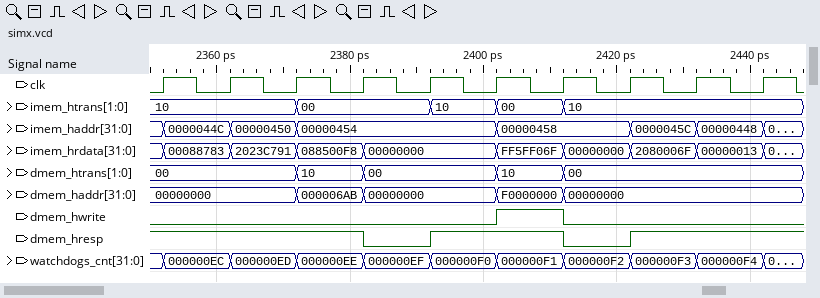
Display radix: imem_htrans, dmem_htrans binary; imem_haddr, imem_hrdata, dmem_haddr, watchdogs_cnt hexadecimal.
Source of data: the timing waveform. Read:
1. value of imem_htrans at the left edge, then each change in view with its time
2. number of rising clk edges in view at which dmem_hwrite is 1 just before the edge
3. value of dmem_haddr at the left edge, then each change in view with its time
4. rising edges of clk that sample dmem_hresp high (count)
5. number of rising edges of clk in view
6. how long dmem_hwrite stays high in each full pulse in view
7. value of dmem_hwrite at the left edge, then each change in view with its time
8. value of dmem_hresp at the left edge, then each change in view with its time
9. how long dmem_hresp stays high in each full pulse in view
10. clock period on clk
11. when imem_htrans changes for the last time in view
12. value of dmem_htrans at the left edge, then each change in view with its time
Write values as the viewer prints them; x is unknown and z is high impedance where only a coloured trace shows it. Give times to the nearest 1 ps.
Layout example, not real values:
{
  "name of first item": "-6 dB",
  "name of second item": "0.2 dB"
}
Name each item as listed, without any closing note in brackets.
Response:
{
  "value of imem_htrans at the left edge, then each change in view with its time": "10, 00 at 2372 ps, 10 at 2392 ps, 00 at 2402 ps, 10 at 2412 ps",
  "number of rising clk edges in view at which dmem_hwrite is 1 just before the edge": "1",
  "value of dmem_haddr at the left edge, then each change in view with its time": "00000000, 000006AB at 2372 ps, 00000000 at 2382 ps, F0000000 at 2402 ps, 00000000 at 2412 ps",
  "rising edges of clk that sample dmem_hresp high": "8",
  "number of rising edges of clk in view": "10",
  "how long dmem_hwrite stays high in each full pulse in view": "10 ps",
  "value of dmem_hwrite at the left edge, then each change in view with its time": "0, 1 at 2402 ps, 0 at 2412 ps",
  "value of dmem_hresp at the left edge, then each change in view with its time": "1, 0 at 2382 ps, 1 at 2392 ps, 0 at 2412 ps, 1 at 2422 ps",
  "how long dmem_hresp stays high in each full pulse in view": "20 ps",
  "clock period on clk": "10 ps",
  "when imem_htrans changes for the last time in view": "2412 ps",
  "value of dmem_htrans at the left edge, then each change in view with its time": "00, 10 at 2372 ps, 00 at 2382 ps, 10 at 2402 ps, 00 at 2412 ps"
}
